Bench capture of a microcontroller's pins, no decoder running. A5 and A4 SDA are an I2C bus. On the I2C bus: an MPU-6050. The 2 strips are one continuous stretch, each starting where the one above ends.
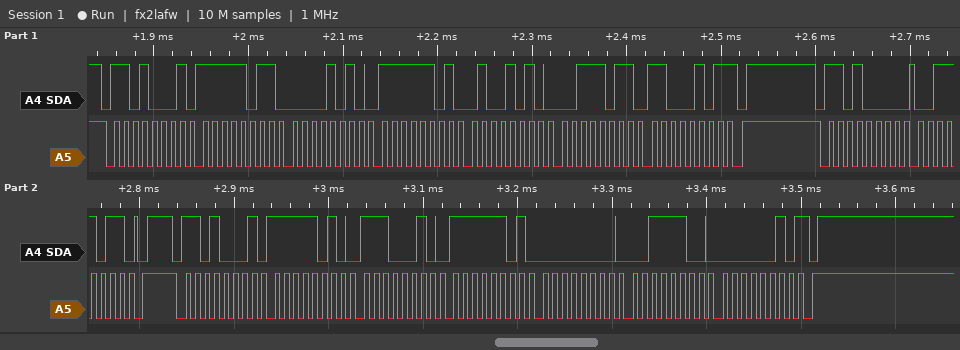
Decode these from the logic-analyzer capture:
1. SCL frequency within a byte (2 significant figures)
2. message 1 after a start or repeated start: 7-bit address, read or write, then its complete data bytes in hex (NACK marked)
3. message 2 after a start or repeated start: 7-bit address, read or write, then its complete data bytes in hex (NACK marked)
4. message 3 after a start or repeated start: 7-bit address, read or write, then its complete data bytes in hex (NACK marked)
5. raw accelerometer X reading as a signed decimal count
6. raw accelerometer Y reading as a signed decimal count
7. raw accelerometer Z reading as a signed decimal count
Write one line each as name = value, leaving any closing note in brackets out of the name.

SCL frequency within a byte = 100 kHz
message 1 after a start or repeated start: 7-bit address, read or write, then its complete data bytes in hex = 0x68 read: FB 0A FD 4A 3B C5 NACK
message 2 after a start or repeated start: 7-bit address, read or write, then its complete data bytes in hex = 0x68 write: 3B
message 3 after a start or repeated start: 7-bit address, read or write, then its complete data bytes in hex = 0x68 read: FA E2 FD 00 3C 02 NACK
raw accelerometer X reading as a signed decimal count = -1310
raw accelerometer Y reading as a signed decimal count = -768
raw accelerometer Z reading as a signed decimal count = 15362
